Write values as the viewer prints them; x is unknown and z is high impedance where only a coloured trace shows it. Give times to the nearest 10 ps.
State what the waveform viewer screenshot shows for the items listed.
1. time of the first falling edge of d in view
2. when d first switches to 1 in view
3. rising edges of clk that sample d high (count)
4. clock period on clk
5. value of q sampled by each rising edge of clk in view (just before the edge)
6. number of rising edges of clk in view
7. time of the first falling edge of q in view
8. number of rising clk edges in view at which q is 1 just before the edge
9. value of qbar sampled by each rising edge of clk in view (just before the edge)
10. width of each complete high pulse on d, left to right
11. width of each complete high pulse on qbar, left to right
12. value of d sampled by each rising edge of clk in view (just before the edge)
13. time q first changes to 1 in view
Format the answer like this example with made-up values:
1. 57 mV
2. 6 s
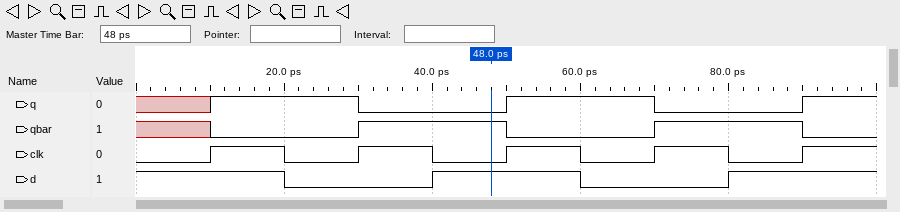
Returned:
1. 20 ps
2. 40 ps
3. 3
4. 20 ps
5. x 1 0 1 0
6. 5
7. 30 ps
8. 2
9. x 0 1 0 1
10. 20 ps
11. 20 ps, 20 ps
12. 1 0 1 0 1
13. 10 ps
